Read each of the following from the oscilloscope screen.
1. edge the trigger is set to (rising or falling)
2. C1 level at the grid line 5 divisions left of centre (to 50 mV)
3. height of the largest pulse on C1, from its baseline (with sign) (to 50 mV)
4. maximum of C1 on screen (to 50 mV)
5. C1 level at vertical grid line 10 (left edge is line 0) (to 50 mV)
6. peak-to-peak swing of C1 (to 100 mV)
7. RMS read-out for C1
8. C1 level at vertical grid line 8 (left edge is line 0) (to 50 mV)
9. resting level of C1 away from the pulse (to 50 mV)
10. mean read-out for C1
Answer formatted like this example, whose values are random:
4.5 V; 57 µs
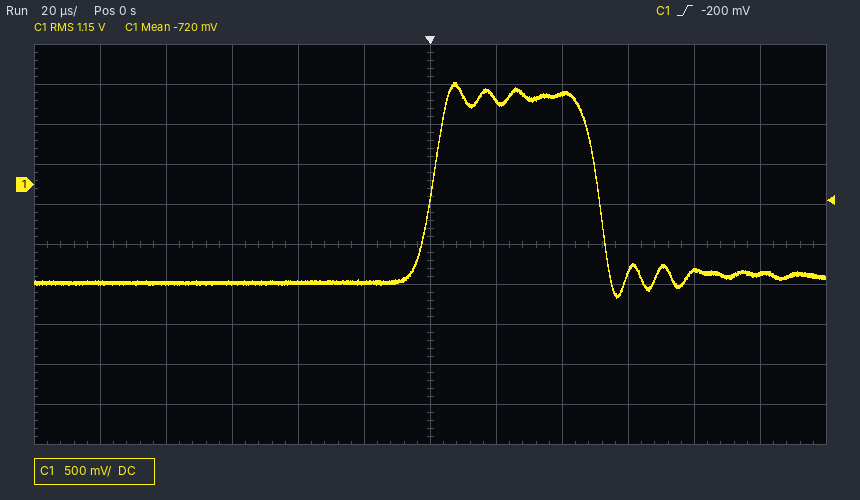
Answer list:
rising; -1.25 V; +2.50 V; 1.25 V; -1.10 V; 2.70 V; 1.15 V; 1.15 V; -1.25 V; -720 mV
